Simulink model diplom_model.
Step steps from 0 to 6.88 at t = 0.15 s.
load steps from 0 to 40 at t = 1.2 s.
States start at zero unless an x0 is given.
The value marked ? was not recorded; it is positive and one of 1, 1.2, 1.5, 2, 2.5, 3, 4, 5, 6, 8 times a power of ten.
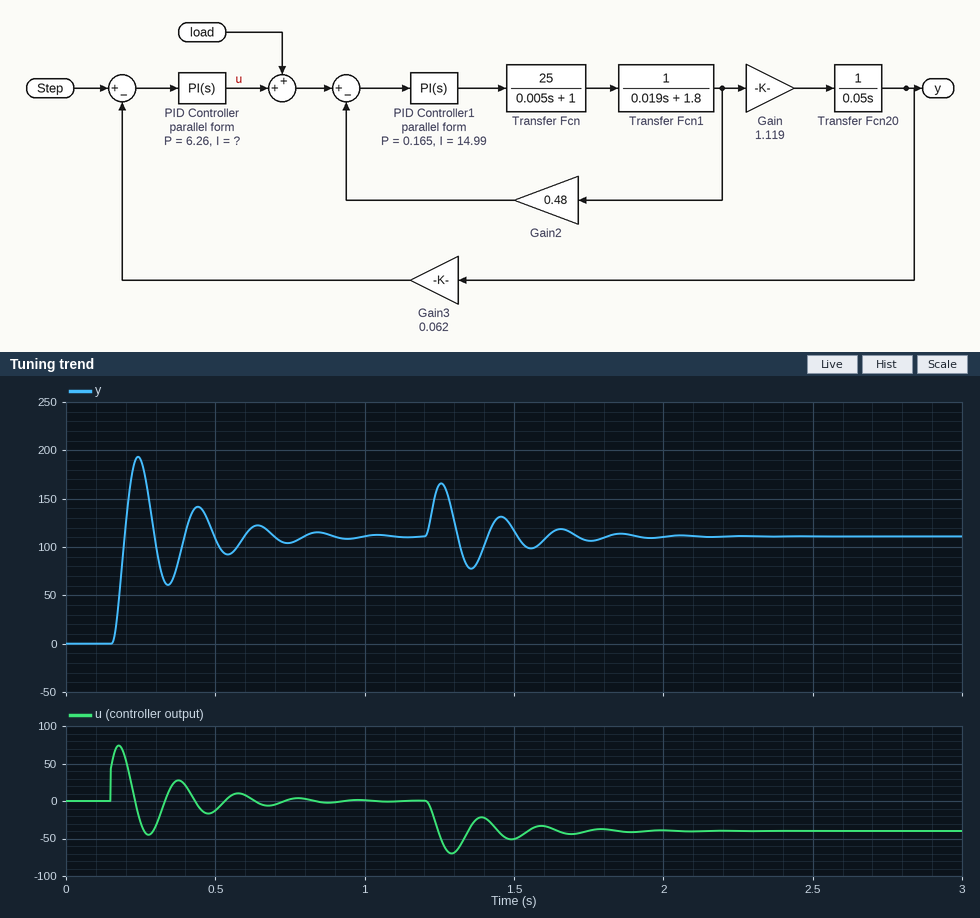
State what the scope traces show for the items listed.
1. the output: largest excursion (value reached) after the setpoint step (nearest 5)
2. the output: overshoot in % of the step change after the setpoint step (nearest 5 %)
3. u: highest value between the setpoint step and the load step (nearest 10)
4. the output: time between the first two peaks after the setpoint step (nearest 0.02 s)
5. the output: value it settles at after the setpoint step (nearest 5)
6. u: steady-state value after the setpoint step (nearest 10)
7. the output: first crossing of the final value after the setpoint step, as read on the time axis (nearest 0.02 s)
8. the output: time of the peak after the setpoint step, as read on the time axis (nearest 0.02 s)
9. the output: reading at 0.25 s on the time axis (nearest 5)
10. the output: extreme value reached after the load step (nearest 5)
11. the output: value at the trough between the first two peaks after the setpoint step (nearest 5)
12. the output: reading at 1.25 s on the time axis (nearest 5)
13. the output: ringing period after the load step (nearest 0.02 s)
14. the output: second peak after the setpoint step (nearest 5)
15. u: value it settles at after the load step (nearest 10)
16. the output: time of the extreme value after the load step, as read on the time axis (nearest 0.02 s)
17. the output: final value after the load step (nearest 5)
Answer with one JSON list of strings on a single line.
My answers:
["195", "75 %", "70", "0.20 s", "110", "0", "0.20 s", "0.24 s", "190", "165", "60", "165", "0.20 s", "140", "-40", "1.26 s", "110"]
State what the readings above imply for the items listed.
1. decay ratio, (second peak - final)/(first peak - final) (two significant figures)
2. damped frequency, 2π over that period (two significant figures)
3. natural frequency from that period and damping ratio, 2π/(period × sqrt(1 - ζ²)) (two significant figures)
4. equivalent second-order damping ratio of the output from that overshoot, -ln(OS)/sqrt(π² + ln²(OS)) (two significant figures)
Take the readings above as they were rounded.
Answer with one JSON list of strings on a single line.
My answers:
["0.35", "31 rad/s", "32 rad/s", "0.091"]
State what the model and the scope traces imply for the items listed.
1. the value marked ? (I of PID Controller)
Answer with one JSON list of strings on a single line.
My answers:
["300"]
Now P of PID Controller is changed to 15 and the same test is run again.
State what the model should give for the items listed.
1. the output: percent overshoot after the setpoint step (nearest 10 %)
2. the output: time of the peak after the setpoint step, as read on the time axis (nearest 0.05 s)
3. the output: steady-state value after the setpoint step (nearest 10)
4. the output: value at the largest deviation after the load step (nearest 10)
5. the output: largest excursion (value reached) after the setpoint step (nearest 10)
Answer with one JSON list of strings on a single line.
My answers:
["40 %", "0.20 s", "110", "150", "160"]
